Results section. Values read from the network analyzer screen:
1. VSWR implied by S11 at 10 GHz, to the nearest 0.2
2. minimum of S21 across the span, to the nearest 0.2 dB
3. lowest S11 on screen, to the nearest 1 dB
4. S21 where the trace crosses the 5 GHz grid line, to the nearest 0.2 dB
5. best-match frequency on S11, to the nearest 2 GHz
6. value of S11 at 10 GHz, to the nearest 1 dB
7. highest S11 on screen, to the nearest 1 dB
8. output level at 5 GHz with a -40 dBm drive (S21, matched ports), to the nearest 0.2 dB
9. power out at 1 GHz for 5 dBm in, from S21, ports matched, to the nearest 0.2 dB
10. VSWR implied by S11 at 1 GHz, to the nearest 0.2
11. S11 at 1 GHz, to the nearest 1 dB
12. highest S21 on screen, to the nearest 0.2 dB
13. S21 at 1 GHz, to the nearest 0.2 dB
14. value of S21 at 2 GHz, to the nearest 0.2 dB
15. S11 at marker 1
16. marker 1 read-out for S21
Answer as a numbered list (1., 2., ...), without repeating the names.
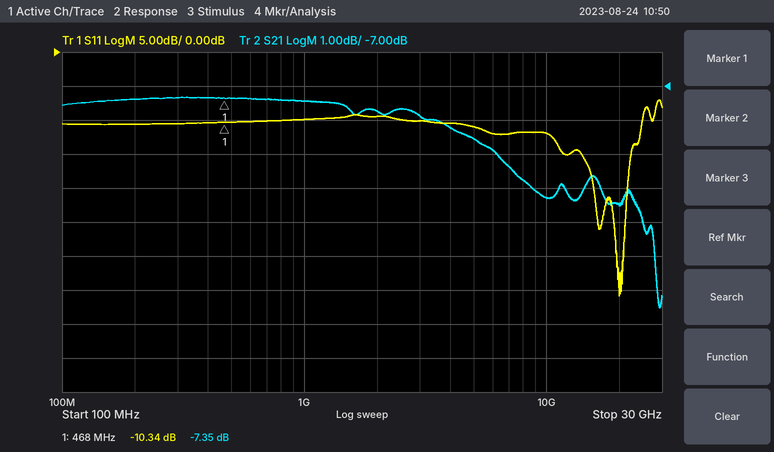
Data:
1. 1.6
2. -13.6 dB
3. -36 dB
4. -8.6 dB
5. 20 GHz
6. -12 dB
7. -7 dB
8. -48.6 dBm
9. -2.4 dBm
10. 2.0
11. -10 dB
12. -7.4 dB
13. -7.4 dB
14. -7.8 dB
15. -10.34 dB
16. -7.35 dB
